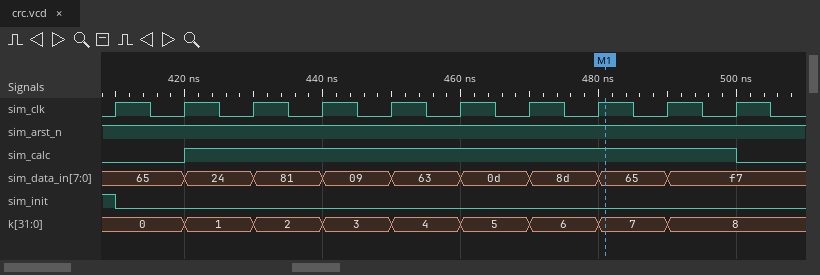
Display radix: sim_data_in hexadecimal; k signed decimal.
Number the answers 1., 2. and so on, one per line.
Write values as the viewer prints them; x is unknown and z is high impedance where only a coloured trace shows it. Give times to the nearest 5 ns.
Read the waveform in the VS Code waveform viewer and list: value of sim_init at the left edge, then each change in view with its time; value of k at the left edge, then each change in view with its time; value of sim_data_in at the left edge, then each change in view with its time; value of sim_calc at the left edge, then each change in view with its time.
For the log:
1. 1, 0 at 410 ns
2. 0, 1 at 420 ns, 2 at 430 ns, 3 at 440 ns, 4 at 450 ns, 5 at 460 ns, 6 at 470 ns, 7 at 480 ns, 8 at 490 ns
3. 65, 24 at 420 ns, 81 at 430 ns, 09 at 440 ns, 63 at 450 ns, 0d at 460 ns, 8d at 470 ns, 65 at 480 ns, f7 at 490 ns
4. 0, 1 at 420 ns, 0 at 500 ns
